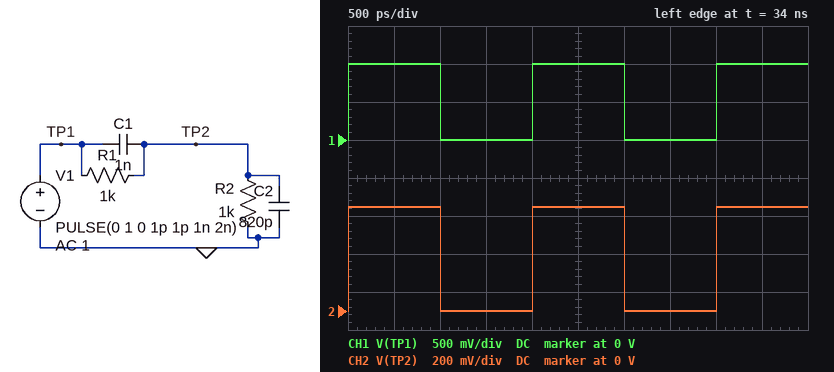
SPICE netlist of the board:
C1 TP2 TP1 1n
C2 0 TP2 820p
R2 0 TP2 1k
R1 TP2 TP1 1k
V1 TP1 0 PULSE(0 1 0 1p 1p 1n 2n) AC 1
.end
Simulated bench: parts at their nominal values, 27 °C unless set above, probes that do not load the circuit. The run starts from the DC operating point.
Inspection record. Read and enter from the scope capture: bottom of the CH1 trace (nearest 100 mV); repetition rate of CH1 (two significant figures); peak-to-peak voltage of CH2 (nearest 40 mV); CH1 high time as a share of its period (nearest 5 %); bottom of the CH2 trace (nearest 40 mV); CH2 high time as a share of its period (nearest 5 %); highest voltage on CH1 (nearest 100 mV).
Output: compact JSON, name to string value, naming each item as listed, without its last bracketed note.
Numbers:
{"bottom of the CH1 trace": "0 V", "repetition rate of CH1": "500 MHz", "peak-to-peak voltage of CH2": "560 mV", "CH1 high time as a share of its period": "50 %", "bottom of the CH2 trace": "0 V", "CH2 high time as a share of its period": "50 %", "highest voltage on CH1": "1.0 V"}
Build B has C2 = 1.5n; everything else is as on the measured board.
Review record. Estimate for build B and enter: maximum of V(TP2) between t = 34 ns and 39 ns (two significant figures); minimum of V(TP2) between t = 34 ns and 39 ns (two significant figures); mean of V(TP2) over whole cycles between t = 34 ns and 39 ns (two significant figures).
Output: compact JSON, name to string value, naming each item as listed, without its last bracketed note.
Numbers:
{"maximum of V(TP2) between t = 34 ns and 39 ns": "400 mV", "minimum of V(TP2) between t = 34 ns and 39 ns": "1.3 mV", "mean of V(TP2) over whole cycles between t = 34 ns and 39 ns": "200 mV"}
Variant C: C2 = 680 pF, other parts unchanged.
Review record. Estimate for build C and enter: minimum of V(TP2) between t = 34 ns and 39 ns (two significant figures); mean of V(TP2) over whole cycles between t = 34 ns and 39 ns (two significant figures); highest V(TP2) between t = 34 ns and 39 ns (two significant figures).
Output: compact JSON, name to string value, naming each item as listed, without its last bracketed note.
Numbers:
{"minimum of V(TP2) between t = 34 ns and 39 ns": "-2.1 mV", "mean of V(TP2) over whole cycles between t = 34 ns and 39 ns": "300 mV", "highest V(TP2) between t = 34 ns and 39 ns": "590 mV"}
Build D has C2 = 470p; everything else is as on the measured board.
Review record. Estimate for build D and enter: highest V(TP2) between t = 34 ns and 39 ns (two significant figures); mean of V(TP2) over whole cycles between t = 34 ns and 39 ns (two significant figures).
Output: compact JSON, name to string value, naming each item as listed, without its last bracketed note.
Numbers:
{"highest V(TP2) between t = 34 ns and 39 ns": "680 mV", "mean of V(TP2) over whole cycles between t = 34 ns and 39 ns": "340 mV"}
